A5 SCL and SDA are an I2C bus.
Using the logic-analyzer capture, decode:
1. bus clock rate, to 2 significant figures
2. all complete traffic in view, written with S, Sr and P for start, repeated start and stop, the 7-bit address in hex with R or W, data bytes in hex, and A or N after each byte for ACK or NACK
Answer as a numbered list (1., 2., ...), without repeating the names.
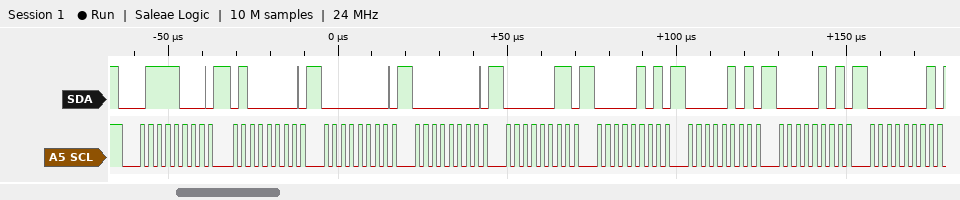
1. 400 kHz
2. S 3CW A 40 A 00 A 00 A 03 A 05 A 05 A 05 A 01 A
